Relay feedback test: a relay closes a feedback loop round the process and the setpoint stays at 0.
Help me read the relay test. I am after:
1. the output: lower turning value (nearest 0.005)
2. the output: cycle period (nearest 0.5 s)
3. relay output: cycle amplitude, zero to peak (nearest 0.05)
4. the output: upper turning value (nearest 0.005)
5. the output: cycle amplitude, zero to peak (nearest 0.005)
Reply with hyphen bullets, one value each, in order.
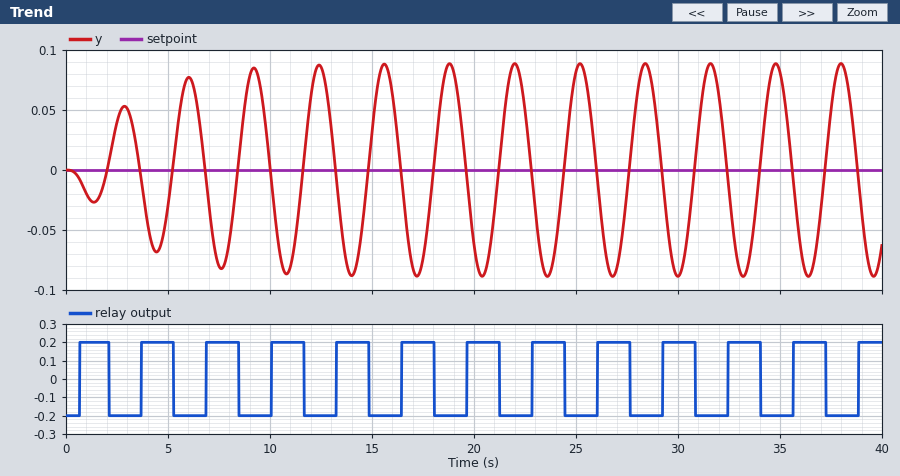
- -0.090
- 3.0 s
- 0.20
- 0.090
- 0.090
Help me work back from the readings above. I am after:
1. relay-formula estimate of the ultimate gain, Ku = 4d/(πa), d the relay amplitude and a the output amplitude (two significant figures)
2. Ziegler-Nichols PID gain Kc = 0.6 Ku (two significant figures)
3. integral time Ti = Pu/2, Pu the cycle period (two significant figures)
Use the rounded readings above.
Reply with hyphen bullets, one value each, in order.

- 2.8
- 1.7
- 1.5 s
